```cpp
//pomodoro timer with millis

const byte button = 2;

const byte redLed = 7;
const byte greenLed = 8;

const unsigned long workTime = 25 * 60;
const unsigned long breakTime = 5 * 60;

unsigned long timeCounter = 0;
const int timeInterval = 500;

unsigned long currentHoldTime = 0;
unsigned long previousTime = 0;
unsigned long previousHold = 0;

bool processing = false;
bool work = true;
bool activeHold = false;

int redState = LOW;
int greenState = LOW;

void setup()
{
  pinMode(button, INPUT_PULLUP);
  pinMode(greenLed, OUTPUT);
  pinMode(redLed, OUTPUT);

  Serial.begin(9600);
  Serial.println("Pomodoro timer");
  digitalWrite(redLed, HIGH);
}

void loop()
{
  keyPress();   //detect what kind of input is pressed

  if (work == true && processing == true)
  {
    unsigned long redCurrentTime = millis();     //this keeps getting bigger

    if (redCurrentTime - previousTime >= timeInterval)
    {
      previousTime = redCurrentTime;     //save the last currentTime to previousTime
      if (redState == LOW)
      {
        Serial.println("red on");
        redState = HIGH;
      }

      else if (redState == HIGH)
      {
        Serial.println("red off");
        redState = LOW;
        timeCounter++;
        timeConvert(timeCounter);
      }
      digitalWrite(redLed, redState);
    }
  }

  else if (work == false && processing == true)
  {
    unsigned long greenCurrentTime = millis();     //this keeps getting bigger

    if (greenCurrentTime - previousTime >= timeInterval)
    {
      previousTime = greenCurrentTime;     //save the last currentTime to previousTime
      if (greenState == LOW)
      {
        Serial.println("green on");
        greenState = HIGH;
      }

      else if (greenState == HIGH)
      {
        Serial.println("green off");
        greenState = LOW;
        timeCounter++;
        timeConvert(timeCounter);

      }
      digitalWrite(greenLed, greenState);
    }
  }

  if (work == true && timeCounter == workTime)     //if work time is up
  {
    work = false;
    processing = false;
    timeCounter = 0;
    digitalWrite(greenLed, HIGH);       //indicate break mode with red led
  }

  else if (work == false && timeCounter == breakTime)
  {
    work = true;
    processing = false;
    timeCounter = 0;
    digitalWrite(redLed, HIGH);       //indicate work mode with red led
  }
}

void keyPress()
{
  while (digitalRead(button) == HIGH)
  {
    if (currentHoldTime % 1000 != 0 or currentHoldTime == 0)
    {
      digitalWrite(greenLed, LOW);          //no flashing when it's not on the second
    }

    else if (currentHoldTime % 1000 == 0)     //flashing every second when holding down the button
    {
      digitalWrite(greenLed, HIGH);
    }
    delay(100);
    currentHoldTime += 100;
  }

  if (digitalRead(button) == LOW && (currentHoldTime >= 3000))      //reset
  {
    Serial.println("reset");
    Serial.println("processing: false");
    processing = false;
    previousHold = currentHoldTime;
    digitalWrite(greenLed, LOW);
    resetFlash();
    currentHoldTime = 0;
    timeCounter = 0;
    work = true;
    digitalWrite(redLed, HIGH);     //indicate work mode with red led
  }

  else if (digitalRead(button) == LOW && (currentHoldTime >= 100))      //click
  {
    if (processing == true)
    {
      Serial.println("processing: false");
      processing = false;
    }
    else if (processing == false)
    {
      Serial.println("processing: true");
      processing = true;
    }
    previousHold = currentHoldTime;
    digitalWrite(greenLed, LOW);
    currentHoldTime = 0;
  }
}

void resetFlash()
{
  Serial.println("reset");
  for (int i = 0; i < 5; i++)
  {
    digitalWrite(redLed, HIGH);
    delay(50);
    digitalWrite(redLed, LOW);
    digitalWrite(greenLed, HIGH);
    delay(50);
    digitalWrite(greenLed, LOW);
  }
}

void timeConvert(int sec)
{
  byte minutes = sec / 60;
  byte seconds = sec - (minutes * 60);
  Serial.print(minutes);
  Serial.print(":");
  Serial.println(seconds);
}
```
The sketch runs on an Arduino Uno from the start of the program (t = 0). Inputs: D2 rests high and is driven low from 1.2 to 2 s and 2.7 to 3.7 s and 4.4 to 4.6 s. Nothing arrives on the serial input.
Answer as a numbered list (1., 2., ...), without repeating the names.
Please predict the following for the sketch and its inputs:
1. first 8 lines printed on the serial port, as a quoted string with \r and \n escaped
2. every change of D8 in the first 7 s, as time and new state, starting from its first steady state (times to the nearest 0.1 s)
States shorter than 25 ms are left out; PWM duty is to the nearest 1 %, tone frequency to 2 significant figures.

1. "Pomodoro timer\r\nprocessing: true\r\nred on\r\nred off\r\n0:1\r\nprocessing: false\r\nprocessing: true\r\nred on\r\n"
2. 0 s low; 1 s high; 1.1 s low; 5.6 s high; 5.7 s low; 6.6 s high; 6.7 s low
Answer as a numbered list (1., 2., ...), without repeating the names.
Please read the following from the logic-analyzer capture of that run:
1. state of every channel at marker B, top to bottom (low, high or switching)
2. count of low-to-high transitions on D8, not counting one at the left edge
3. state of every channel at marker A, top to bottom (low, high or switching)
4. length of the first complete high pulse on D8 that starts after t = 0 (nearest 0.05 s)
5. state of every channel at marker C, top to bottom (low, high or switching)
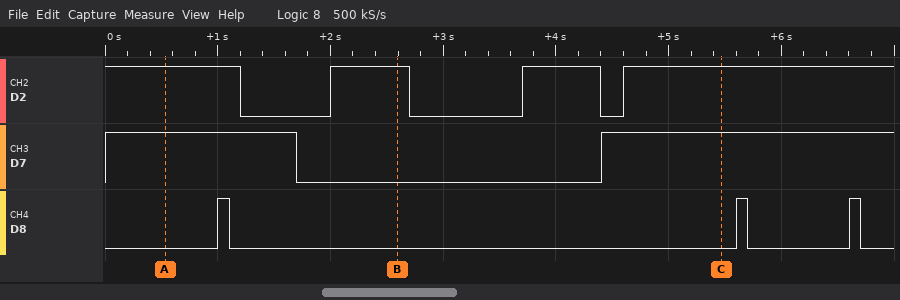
1. D2 high, D7 low, D8 low
2. 3
3. D2 high, D7 high, D8 low
4. 0.10 s
5. D2 high, D7 high, D8 low
